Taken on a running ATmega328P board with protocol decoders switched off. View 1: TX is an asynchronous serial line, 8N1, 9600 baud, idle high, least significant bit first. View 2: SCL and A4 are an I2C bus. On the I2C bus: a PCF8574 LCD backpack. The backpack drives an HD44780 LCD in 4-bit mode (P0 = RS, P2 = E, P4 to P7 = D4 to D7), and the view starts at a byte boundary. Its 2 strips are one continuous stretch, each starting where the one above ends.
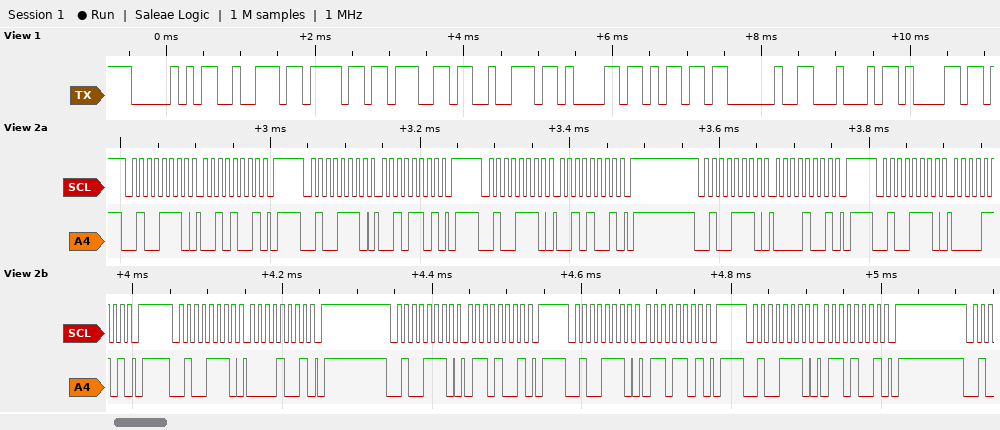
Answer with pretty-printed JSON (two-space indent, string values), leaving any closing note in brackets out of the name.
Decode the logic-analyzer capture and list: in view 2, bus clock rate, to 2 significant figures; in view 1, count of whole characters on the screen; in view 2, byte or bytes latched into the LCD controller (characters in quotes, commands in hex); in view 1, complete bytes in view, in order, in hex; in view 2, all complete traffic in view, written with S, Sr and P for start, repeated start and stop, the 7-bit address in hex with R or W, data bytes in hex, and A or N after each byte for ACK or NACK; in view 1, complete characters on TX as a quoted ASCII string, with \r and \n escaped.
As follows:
{
  "in view 2, bus clock rate, to 2 significant figures": "100 kHz",
  "in view 1, count of whole characters on the screen": "10",
  "in view 2, byte or bytes latched into the LCD controller": "' '",
  "in view 1, complete bytes in view, in order, in hex": "50 72 6F 67 72 61 6D 20 44 61",
  "in view 2, all complete traffic in view, written with S, Sr and P for start, repeated start and stop, the 7-bit address in hex with R or W, data bytes in hex, and A or N after each byte for ACK or NACK": "S 27W A 29 A P S 27W A 2D A P S 27W A 29 A P S 27W A 09 A P S 27W A 0D A P S 27W A 09 A P S 27W A 69 A P S 27W A 6D A P S 27W A 69 A P",
  "in view 1, complete characters on TX as a quoted ASCII string, with \\r and \\n escaped": "\"Program Da\""
}
